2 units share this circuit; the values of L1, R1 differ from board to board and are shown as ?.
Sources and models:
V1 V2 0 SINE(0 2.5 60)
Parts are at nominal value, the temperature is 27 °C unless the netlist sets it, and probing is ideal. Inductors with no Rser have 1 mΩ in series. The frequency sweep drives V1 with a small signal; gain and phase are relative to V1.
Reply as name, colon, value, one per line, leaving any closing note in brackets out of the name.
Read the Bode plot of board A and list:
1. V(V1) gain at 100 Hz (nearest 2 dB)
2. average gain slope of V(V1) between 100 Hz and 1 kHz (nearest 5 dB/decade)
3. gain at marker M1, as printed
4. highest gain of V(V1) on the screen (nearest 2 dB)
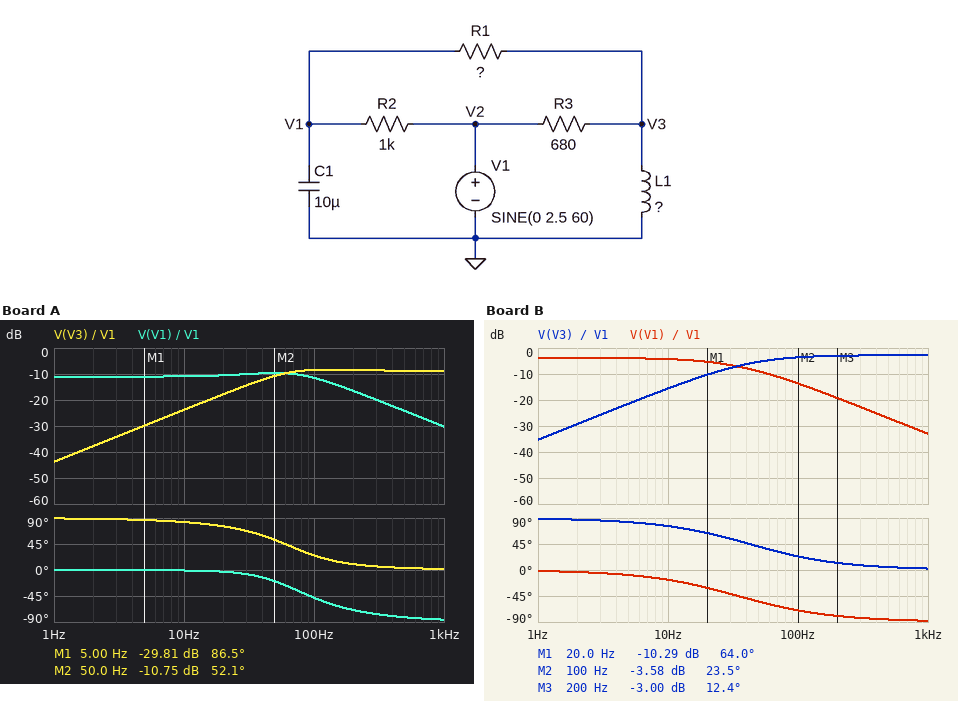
V(V1) gain at 100 Hz: -12 dB
average gain slope of V(V1) between 100 Hz and 1 kHz: -20 dB/decade
gain at marker M1, as printed: -29.81 dB
highest gain of V(V1) on the screen: -10 dB
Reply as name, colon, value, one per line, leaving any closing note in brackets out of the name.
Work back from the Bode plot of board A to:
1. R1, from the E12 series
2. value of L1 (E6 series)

R1, from the E12 series: 390 Ω
value of L1: 470 mH
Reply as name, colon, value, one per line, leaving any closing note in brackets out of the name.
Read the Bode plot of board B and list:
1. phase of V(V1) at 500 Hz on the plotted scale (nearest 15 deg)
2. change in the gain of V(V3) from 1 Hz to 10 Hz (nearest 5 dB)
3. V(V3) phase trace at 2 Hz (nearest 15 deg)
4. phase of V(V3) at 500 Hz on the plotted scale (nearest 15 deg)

phase of V(V1) at 500 Hz on the plotted scale: -90 deg
change in the gain of V(V3) from 1 Hz to 10 Hz: 20 dB
V(V3) phase trace at 2 Hz: 90 deg
phase of V(V3) at 500 Hz on the plotted scale: 0 deg
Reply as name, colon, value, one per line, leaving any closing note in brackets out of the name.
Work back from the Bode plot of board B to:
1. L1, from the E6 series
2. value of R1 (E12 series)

L1, from the E6 series: 1.5 H
value of R1: 1.8 kΩ
